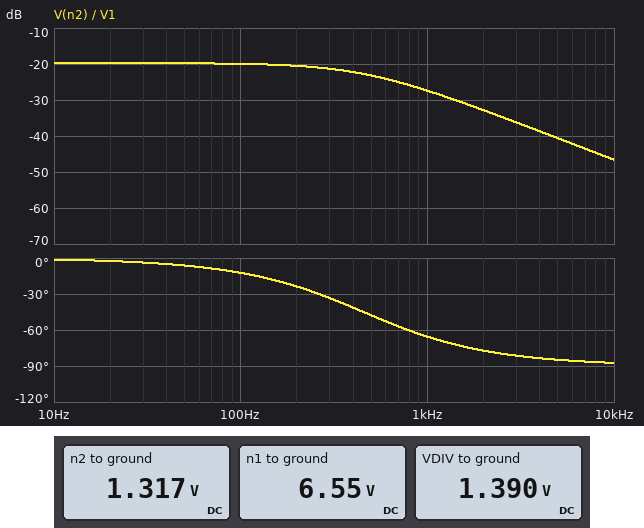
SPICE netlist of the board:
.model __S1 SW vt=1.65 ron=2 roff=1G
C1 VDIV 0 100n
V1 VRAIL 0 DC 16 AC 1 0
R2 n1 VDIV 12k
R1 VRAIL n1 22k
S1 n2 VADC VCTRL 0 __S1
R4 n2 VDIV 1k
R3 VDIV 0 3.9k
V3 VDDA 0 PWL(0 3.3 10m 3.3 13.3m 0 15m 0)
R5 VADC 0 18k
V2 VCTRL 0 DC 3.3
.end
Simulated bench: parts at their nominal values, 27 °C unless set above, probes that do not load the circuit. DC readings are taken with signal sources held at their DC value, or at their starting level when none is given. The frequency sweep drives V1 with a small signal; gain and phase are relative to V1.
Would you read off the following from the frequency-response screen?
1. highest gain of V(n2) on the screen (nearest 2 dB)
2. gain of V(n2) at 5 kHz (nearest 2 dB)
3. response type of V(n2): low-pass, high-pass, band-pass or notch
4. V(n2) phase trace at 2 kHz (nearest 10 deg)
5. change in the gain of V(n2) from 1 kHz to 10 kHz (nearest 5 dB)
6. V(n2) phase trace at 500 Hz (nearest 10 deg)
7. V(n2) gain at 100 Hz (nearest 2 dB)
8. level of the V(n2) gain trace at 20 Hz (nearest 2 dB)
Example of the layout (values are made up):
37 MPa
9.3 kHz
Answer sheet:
-20 dB
-40 dB
low-pass
-80 deg
-20 dB
-50 deg
-20 dB
-20 dB
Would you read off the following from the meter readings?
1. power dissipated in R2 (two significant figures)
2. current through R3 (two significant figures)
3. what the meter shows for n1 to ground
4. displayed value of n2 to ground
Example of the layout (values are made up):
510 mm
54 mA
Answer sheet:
2.2 mW
360 µA
6.55 V
1.317 V
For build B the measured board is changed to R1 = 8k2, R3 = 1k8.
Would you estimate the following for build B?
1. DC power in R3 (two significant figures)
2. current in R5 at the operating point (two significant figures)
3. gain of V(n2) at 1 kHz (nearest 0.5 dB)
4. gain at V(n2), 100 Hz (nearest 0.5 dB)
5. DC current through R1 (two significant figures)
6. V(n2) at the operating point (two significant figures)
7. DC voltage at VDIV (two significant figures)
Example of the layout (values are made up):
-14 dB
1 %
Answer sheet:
810 µW
63 µA
-25.0 dB
-22.0 dB
730 µA
1.1 V
1.2 V
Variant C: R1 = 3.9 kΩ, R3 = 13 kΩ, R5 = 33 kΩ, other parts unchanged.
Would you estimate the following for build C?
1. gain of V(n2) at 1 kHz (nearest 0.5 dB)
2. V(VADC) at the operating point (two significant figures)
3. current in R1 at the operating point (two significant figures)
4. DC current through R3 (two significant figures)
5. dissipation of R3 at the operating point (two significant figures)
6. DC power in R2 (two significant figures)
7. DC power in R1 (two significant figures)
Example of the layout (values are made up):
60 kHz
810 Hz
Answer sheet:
-20.0 dB
5.8 V
630 µA
460 µA
2.7 mW
4.8 mW
1.6 mW
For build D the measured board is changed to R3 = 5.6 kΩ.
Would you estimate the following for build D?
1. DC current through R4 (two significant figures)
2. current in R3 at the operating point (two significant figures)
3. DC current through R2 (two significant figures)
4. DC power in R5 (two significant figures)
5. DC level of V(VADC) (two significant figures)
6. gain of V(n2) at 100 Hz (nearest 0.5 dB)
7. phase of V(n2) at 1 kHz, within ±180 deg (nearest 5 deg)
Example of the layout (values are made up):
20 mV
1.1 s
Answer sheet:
95 µA
320 µA
420 µA
160 µW
1.7 V
-17.5 dB
-70 deg
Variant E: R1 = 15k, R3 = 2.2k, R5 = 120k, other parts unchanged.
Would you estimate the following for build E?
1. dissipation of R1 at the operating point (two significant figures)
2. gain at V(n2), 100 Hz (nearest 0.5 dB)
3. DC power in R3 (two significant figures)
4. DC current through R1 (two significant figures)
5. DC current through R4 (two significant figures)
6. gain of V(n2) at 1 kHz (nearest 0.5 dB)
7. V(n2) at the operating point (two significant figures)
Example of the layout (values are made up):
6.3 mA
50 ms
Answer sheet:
4.5 mW
-22.5 dB
640 µW
550 µA
9.8 µA
-26.5 dB
1.2 V
